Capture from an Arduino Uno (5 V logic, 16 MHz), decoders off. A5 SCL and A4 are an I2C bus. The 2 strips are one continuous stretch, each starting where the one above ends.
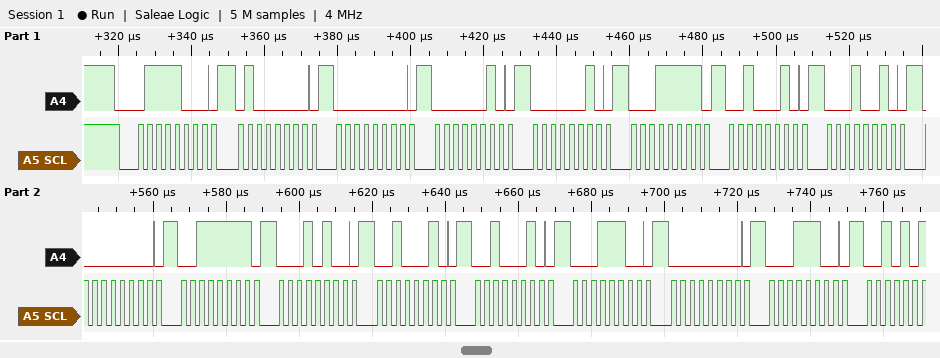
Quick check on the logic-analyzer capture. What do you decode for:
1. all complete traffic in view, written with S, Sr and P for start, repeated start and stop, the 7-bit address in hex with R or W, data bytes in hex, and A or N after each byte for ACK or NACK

S 3CW A 40 A 00 A 02 A 02 A 1F A 22 A 12 A 00 A 3F A 14 A 22 A 22 A 1C A 00 A 1C A
